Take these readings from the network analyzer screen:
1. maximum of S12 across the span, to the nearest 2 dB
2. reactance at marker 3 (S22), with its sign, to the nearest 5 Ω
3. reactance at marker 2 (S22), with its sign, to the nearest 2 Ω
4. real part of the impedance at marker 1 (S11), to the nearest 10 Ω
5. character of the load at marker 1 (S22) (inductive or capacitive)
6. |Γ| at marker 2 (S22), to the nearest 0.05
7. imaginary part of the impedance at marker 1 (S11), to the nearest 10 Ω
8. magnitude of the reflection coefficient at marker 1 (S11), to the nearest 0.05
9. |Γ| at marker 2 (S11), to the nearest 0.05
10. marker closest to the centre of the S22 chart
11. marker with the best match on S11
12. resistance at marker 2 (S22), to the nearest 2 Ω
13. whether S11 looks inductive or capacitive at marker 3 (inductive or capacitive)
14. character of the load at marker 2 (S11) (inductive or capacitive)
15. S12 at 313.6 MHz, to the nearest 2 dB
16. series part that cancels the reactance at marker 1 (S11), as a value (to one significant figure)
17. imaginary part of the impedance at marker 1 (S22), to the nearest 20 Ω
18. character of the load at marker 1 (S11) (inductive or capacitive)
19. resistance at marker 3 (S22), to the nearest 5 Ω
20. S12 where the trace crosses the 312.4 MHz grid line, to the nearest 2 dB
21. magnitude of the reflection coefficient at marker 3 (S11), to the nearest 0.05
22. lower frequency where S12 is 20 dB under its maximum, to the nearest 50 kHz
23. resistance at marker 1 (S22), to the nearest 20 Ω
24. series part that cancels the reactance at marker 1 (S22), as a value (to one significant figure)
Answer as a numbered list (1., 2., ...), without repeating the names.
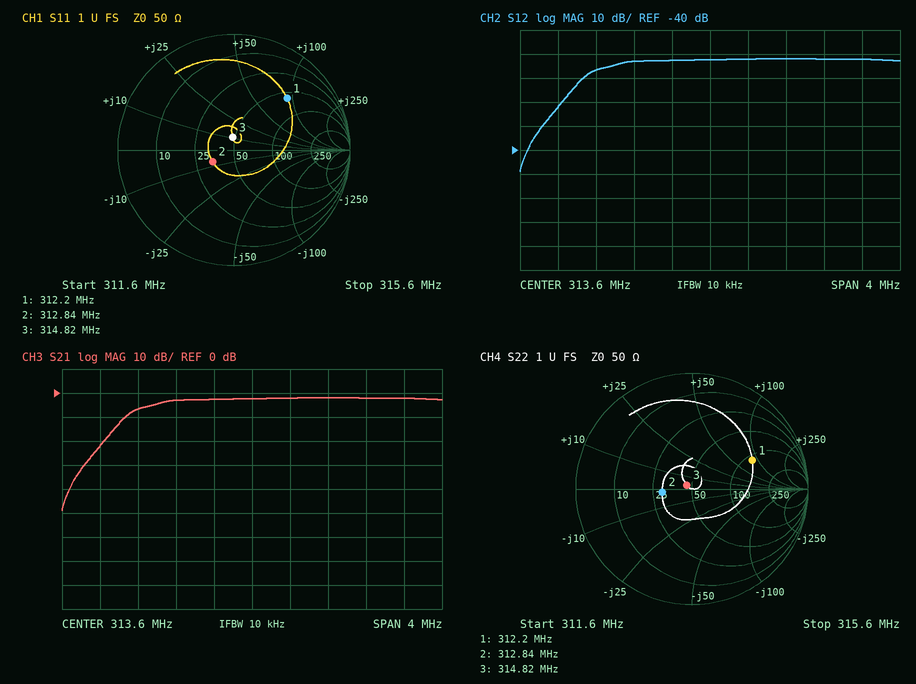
1. -2 dB
2. +5 Ω
3. -2 Ω
4. 60 Ω
5. inductive
6. 0.25
7. +90 Ω
8. 0.65
9. 0.20
10. marker 3
11. marker 3
12. 30 Ω
13. inductive
14. capacitive
15. -2 dB
16. 6 pF
17. +80 Ω
18. inductive
19. 45 Ω
20. -6 dB
21. 0.10
22. 312.00 MHz
23. 120 Ω
24. 6 pF
